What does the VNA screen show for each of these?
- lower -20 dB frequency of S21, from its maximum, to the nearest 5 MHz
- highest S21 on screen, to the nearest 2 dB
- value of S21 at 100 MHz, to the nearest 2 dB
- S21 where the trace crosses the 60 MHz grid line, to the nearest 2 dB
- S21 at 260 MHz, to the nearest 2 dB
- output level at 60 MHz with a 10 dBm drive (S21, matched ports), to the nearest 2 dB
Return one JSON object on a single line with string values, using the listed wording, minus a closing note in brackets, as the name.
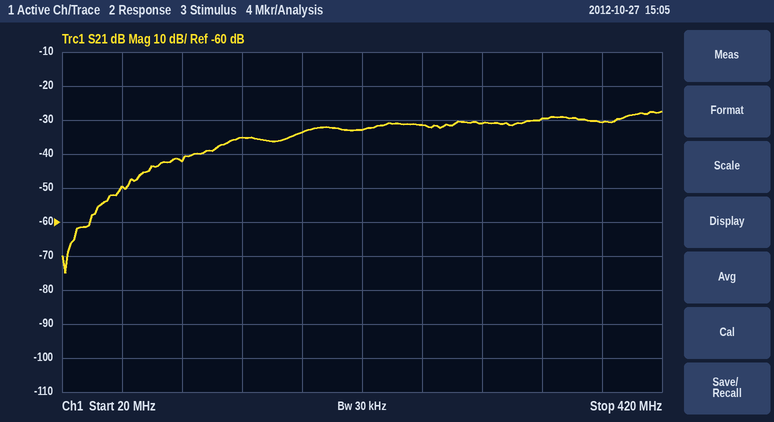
{"lower -20 dB frequency of S21, from its maximum, to the nearest 5 MHz": "70 MHz", "highest S21 on screen, to the nearest 2 dB": "-28 dB", "value of S21 at 100 MHz, to the nearest 2 dB": "-42 dB", "S21 where the trace crosses the 60 MHz grid line, to the nearest 2 dB": "-50 dB", "S21 at 260 MHz, to the nearest 2 dB": "-32 dB", "output level at 60 MHz with a 10 dBm drive (S21, matched ports), to the nearest 2 dB": "-40 dBm"}
